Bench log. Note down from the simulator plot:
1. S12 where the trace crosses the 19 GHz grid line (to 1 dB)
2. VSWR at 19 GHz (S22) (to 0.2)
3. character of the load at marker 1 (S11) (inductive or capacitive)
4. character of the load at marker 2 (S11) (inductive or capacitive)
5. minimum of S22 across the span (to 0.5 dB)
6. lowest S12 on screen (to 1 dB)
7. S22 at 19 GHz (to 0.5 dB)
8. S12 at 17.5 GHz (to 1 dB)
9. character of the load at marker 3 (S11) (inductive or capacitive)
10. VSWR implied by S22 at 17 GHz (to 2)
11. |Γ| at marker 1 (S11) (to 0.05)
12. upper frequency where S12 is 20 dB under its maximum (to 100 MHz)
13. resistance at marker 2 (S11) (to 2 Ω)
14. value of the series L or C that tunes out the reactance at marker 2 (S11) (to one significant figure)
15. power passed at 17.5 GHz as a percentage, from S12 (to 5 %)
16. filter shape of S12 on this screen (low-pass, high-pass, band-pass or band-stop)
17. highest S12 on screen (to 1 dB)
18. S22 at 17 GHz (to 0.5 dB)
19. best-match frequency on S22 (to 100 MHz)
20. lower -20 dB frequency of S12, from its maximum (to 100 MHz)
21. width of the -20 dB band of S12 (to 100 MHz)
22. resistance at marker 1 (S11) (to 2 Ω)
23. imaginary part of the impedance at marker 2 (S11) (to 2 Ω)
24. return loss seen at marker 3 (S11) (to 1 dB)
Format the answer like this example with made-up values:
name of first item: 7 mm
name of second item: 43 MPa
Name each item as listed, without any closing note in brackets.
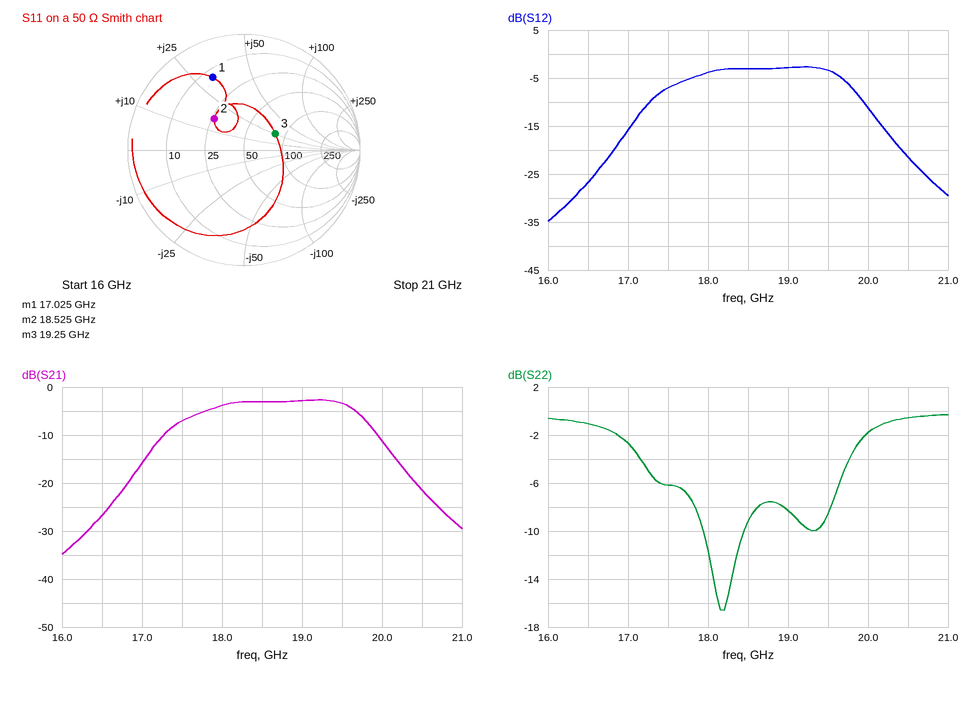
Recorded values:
S12 where the trace crosses the 19 GHz grid line: -3 dB
VSWR at 19 GHz (S22): 2.2
character of the load at marker 1 (S11): inductive
character of the load at marker 2 (S11): inductive
minimum of S22 across the span: -16.5 dB
lowest S12 on screen: -35 dB
S22 at 19 GHz: -8.5 dB
S12 at 17.5 GHz: -7 dB
character of the load at marker 3 (S11): inductive
VSWR implied by S22 at 17 GHz: 6
|Γ| at marker 1 (S11): 0.70
upper frequency where S12 is 20 dB under its maximum: 20.6 GHz
resistance at marker 2 (S11): 26 Ω
value of the series L or C that tunes out the reactance at marker 2 (S11): 500 fF
power passed at 17.5 GHz as a percentage, from S12: 20 %
filter shape of S12 on this screen: band-pass
highest S12 on screen: -3 dB
S22 at 17 GHz: -2.5 dB
best-match frequency on S22: 18.2 GHz
lower -20 dB frequency of S12, from its maximum: 16.7 GHz
width of the -20 dB band of S12: 3.9 GHz
resistance at marker 1 (S11): 14 Ω
imaginary part of the impedance at marker 2 (S11): +16 Ω
return loss seen at marker 3 (S11): 10 dB
